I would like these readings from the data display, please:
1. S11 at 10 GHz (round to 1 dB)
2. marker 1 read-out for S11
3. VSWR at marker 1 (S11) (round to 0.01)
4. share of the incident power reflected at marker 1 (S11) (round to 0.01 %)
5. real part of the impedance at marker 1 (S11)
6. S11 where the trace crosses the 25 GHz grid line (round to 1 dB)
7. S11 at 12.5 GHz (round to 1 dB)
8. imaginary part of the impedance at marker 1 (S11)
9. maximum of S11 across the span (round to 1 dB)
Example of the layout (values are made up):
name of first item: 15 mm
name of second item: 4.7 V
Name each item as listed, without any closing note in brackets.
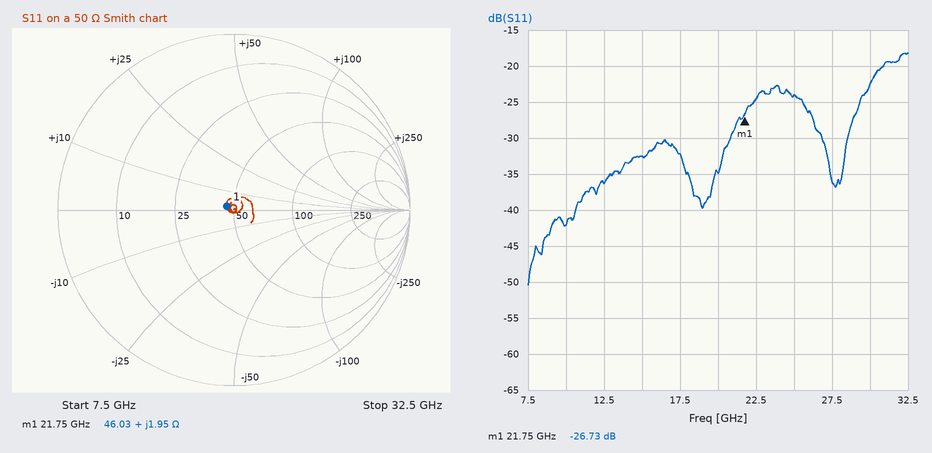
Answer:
S11 at 10 GHz: -42 dB
marker 1 read-out for S11: -26.73 dB
VSWR at marker 1 (S11): 1.10
share of the incident power reflected at marker 1 (S11): 0.21 %
real part of the impedance at marker 1: 46.03 Ω
S11 where the trace crosses the 25 GHz grid line: -24 dB
S11 at 12.5 GHz: -36 dB
imaginary part of the impedance at marker 1: +1.95 Ω
maximum of S11 across the span: -18 dB
